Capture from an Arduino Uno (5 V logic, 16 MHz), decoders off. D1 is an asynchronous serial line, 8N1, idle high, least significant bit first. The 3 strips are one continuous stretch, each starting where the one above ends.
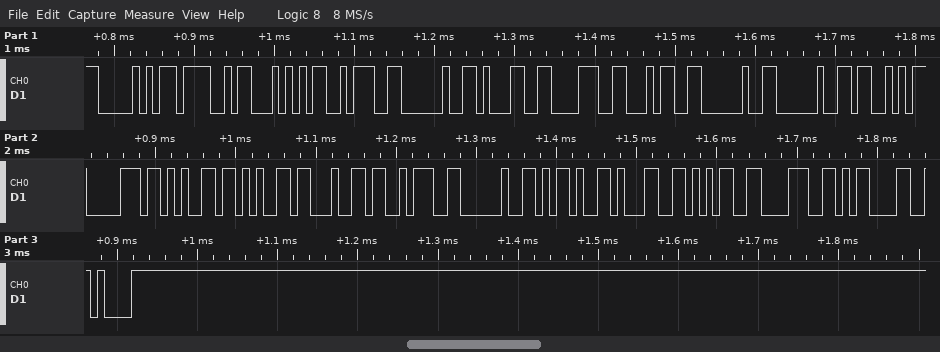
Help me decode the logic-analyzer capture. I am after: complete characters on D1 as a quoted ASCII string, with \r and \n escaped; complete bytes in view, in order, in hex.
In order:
"POT: 184  Speed: -158\r\n"
50 4F 54 3A 20 31 38 34 20 20 53 70 65 65 64 3A 20 2D 31 35 38 0D 0A
